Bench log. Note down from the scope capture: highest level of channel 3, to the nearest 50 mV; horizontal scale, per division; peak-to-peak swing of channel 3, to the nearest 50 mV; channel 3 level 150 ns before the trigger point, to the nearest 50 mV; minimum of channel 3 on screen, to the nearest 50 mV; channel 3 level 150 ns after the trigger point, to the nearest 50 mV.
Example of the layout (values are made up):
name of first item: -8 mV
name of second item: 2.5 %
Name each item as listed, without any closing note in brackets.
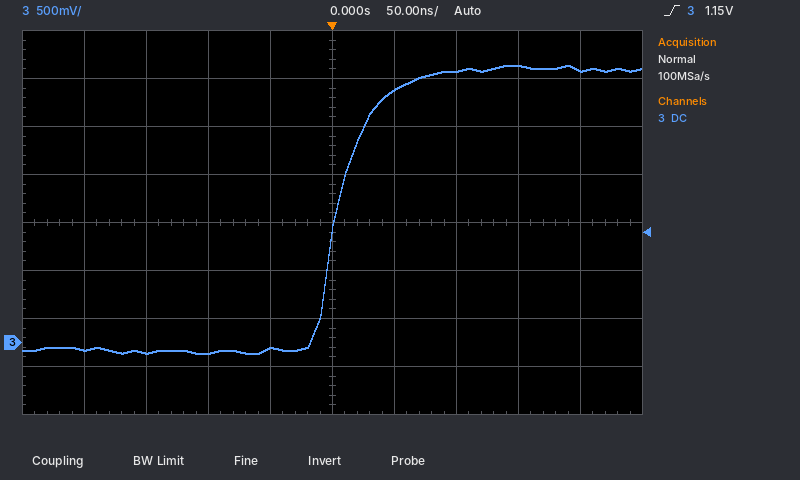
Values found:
highest level of channel 3, to the nearest 50 mV: 2.90 V
horizontal scale, per division: 50 ns
peak-to-peak swing of channel 3, to the nearest 50 mV: 3.00 V
channel 3 level 150 ns before the trigger point, to the nearest 50 mV: -100 mV
minimum of channel 3 on screen, to the nearest 50 mV: -100 mV
channel 3 level 150 ns after the trigger point, to the nearest 50 mV: 2.90 V
